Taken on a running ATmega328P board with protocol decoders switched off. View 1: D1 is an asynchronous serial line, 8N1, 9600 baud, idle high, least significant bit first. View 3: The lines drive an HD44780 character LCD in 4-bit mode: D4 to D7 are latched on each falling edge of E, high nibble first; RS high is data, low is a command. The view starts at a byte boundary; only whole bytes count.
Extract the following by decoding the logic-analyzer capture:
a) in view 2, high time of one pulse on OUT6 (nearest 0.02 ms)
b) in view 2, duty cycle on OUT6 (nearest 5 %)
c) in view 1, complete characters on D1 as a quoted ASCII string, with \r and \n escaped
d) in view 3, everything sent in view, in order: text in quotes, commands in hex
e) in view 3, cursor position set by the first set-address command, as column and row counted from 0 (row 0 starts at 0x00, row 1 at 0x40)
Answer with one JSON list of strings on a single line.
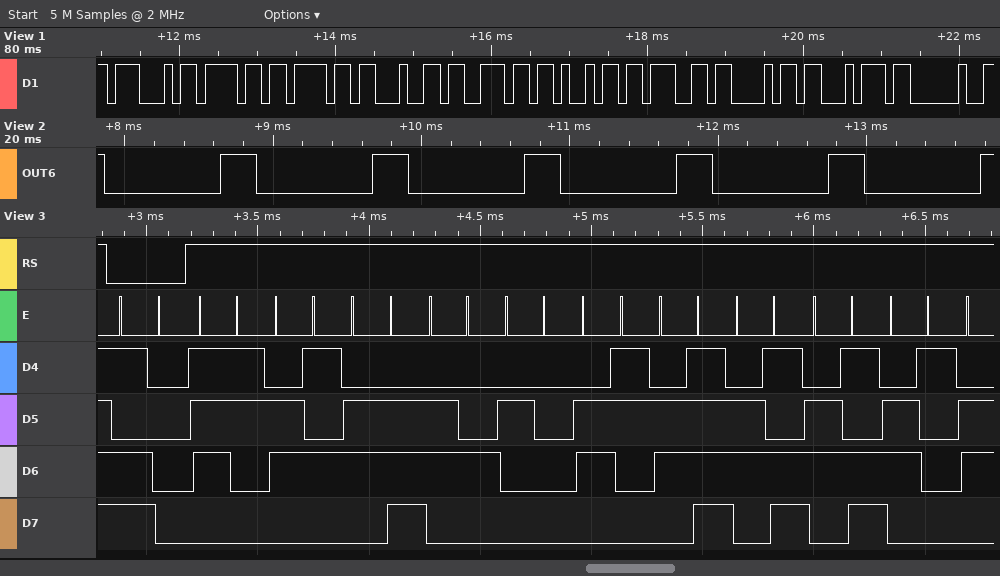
["0.24 ms", "25 %", "\"Goodnight \"", "0xD0 \"send comma\"", "column 16, row 1"]
